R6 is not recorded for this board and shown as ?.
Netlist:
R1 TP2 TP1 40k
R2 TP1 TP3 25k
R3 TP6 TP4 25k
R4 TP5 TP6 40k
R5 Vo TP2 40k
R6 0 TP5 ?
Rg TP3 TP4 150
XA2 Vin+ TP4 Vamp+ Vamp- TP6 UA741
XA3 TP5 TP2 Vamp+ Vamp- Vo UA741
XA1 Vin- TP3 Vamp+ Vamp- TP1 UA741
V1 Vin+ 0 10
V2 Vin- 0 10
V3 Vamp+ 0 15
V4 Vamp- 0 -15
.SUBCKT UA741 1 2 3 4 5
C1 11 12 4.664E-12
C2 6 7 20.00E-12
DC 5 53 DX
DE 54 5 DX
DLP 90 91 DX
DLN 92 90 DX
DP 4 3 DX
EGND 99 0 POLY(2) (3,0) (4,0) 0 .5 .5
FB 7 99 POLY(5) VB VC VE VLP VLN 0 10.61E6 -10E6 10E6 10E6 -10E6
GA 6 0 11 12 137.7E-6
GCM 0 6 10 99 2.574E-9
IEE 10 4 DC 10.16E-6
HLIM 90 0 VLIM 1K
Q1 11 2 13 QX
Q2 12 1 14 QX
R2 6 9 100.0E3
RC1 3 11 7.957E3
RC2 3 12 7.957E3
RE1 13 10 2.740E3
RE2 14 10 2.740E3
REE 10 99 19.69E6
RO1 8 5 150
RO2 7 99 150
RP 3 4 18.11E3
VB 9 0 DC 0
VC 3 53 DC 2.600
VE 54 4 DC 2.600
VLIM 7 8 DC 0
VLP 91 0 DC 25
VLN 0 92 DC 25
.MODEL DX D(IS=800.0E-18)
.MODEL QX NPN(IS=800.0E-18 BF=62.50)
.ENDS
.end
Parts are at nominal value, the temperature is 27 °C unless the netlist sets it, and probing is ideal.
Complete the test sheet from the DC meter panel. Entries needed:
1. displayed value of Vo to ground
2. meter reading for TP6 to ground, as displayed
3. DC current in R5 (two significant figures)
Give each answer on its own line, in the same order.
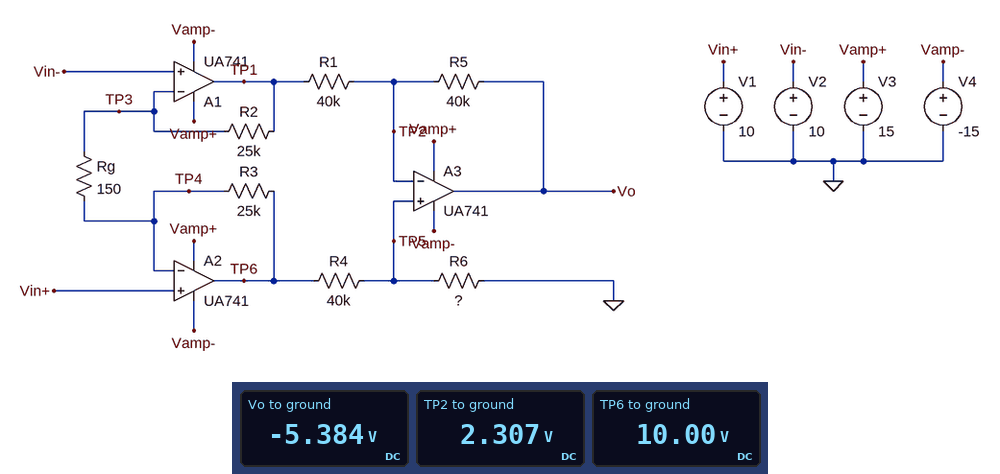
-5.384 V
10.00 V
190 µA
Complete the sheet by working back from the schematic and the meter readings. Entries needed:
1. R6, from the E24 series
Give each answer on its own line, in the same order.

12 kΩ
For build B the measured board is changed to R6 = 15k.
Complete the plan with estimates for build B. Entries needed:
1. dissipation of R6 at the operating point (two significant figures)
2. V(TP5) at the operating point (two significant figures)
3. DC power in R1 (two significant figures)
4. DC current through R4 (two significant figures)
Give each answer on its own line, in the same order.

500 µW
2.7 V
1.3 mW
180 µA
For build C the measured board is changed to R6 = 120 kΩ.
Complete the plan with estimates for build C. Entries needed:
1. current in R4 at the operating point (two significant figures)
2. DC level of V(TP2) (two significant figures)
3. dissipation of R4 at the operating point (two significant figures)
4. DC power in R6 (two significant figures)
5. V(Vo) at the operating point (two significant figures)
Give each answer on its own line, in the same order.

63 µA
7.5 V
160 µW
470 µW
5.0 V
